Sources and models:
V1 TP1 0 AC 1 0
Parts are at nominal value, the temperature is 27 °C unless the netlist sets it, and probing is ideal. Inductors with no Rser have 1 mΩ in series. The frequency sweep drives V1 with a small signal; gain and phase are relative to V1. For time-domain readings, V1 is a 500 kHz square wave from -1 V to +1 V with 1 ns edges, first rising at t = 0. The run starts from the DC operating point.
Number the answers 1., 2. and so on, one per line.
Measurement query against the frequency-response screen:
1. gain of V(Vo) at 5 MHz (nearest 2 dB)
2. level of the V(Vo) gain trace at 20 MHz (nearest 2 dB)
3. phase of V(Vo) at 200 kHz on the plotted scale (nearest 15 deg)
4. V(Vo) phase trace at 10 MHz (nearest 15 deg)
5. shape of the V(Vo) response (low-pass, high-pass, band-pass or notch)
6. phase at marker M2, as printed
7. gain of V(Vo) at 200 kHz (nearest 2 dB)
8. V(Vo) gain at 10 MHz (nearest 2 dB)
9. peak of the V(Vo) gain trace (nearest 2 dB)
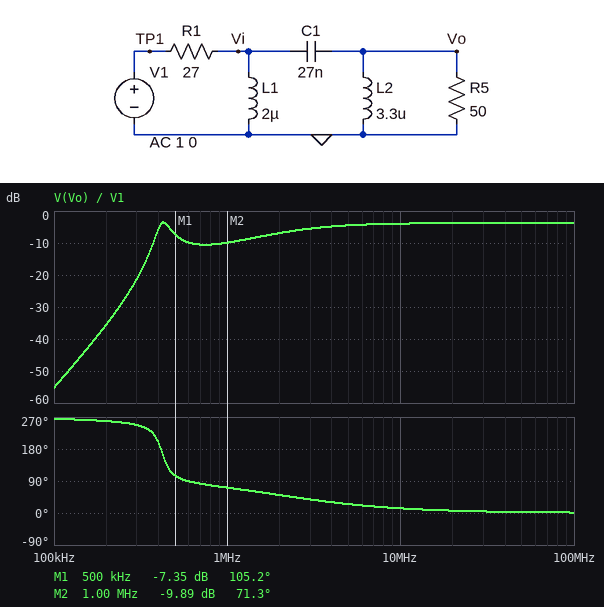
1. -4 dB
2. -4 dB
3. 255 deg
4. 15 deg
5. high-pass
6. 71.3 deg
7. -36 dB
8. -4 dB
9. -4 dB
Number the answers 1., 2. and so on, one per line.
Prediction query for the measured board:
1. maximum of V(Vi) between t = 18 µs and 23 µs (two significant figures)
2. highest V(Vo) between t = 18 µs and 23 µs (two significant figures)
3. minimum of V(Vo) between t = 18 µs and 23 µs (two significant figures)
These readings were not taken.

1. 1.1 V
2. 1.7 V
3. -1.7 V
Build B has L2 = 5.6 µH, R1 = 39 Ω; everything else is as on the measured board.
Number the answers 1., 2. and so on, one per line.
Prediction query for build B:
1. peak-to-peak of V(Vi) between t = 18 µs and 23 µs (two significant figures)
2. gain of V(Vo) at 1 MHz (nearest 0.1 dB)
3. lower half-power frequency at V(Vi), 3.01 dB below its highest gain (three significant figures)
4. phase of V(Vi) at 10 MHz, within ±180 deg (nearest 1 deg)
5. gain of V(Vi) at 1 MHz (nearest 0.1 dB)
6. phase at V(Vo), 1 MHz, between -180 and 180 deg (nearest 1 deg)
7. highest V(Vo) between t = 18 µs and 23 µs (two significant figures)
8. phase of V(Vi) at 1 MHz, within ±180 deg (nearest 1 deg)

1. 2.1 V
2. -12.1 dB
3. 2.39 MHz
4. 13 deg
5. -13.6 dB
6. 72 deg
7. 1.3 V
8. 64 deg
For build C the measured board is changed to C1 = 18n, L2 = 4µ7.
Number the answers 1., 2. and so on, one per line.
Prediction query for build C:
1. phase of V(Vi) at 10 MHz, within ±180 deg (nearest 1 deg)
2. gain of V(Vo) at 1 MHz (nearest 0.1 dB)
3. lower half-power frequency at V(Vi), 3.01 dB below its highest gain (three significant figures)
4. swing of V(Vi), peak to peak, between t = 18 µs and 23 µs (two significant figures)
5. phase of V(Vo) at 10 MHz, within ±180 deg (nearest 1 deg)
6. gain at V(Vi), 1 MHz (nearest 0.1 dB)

1. 11 deg
2. -8.7 dB
3. 2.07 MHz
4. 2.3 V
5. 12 deg
6. -11.6 dB
